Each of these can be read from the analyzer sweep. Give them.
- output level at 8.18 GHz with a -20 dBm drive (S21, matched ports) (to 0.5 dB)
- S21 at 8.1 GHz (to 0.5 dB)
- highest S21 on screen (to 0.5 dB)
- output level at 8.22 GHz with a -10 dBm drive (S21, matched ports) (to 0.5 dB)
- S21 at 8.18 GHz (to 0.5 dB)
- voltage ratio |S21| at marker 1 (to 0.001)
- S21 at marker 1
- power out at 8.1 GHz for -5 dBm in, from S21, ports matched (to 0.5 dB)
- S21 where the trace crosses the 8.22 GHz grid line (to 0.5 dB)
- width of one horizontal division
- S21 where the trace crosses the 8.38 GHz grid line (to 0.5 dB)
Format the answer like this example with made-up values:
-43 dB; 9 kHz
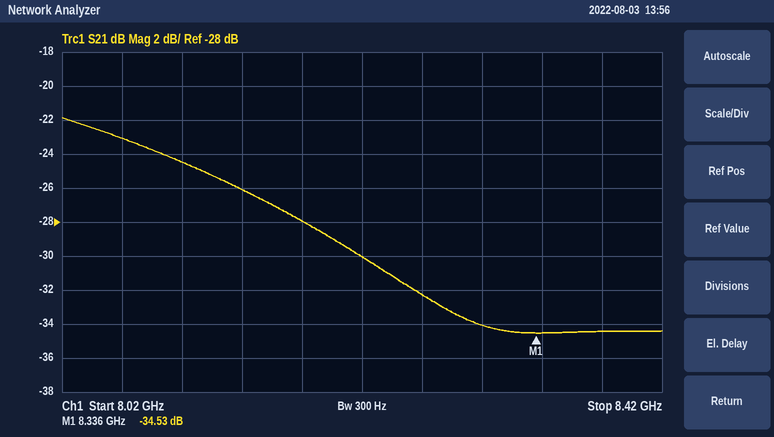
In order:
-48.0 dBm; -24.5 dB; -22.0 dB; -40.0 dBm; -28.0 dB; 0.019; -34.53 dB; -29.5 dBm; -30.0 dB; 40 MHz; -34.5 dB
